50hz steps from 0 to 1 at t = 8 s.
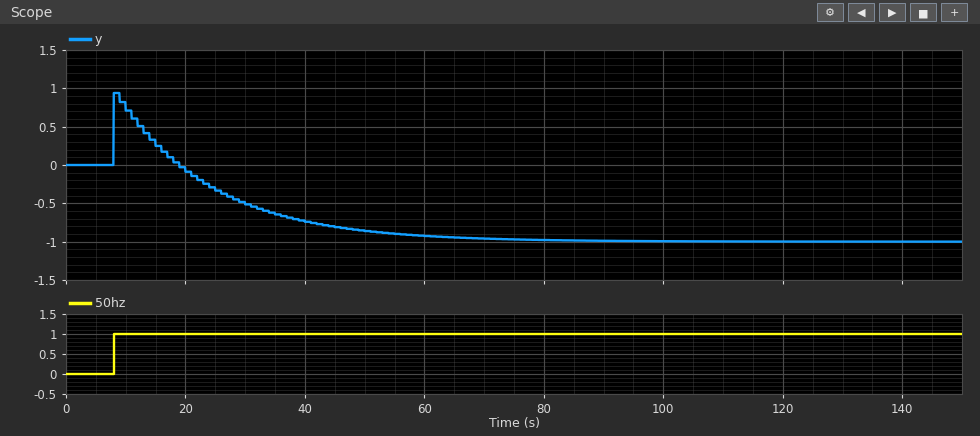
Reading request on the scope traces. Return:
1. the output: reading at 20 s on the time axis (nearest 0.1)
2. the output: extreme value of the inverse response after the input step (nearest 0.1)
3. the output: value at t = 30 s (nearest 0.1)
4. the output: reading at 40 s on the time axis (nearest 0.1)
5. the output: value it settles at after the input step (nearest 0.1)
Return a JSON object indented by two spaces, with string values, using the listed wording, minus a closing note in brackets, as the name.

{
  "the output: reading at 20 s on the time axis": "-0.1",
  "the output: extreme value of the inverse response after the input step": "0.9",
  "the output: value at t = 30 s": "-0.5",
  "the output: reading at 40 s on the time axis": "-0.7",
  "the output: value it settles at after the input step": "-1.0"
}
